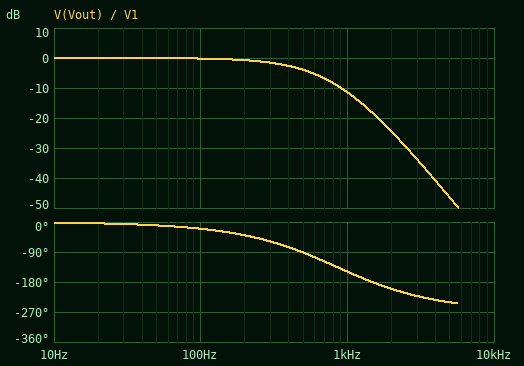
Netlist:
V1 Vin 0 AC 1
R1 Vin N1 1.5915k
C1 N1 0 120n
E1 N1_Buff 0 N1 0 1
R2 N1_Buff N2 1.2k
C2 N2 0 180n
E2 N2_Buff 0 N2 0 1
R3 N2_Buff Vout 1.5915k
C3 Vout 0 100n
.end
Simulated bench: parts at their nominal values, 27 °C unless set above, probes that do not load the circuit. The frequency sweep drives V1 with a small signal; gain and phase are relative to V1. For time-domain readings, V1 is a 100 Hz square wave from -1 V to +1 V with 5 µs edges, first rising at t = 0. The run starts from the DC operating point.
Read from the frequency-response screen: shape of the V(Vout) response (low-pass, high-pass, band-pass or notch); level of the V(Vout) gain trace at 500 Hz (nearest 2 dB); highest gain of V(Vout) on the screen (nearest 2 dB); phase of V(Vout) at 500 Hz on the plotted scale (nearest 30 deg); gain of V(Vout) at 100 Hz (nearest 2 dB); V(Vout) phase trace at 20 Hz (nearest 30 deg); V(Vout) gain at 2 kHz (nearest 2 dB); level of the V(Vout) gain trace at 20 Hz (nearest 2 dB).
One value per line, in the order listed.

low-pass
-4 dB
0 dB
-90 deg
0 dB
0 deg
-24 dB
0 dB
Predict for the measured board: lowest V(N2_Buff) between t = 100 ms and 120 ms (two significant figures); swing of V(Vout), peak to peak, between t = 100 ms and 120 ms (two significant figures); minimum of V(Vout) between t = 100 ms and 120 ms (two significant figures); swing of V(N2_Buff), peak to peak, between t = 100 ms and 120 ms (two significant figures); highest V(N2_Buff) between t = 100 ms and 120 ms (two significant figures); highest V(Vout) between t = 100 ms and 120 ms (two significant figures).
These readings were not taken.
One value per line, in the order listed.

-1.0 V
2.0 V
-1.0 V
2.0 V
1.0 V
1.0 V
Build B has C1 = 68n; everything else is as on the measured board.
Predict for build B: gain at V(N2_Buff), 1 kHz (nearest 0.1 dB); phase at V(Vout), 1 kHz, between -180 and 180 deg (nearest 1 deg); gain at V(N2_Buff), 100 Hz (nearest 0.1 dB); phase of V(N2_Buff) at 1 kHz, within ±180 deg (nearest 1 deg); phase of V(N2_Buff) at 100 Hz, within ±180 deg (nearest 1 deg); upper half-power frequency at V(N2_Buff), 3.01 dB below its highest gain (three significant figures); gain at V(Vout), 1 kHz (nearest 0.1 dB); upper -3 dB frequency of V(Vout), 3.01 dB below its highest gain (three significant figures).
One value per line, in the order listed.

-6.2 dB
-133 deg
-0.1 dB
-88 deg
-12 deg
617 Hz
-9.2 dB
493 Hz
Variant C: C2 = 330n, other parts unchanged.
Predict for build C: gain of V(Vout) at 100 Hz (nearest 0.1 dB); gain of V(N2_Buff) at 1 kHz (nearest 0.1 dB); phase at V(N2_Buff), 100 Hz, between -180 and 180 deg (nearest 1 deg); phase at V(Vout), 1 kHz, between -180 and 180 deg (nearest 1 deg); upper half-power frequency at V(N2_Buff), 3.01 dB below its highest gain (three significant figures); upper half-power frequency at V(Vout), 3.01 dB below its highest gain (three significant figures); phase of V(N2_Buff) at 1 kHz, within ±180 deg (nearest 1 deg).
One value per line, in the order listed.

-0.4 dB
-12.4 dB
-21 deg
-163 deg
340 Hz
311 Hz
-118 deg
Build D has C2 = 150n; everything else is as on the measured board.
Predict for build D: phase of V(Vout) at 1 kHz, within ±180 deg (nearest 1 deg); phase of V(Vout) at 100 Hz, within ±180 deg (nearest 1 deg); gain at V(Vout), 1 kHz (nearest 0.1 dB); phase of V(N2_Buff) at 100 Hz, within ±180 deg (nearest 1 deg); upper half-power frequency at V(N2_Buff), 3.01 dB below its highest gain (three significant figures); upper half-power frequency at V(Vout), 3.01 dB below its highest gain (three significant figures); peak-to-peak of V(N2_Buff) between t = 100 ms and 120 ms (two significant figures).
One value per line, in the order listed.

-144 deg
-19 deg
-10.5 dB
-13 deg
552 Hz
458 Hz
2.0 V
